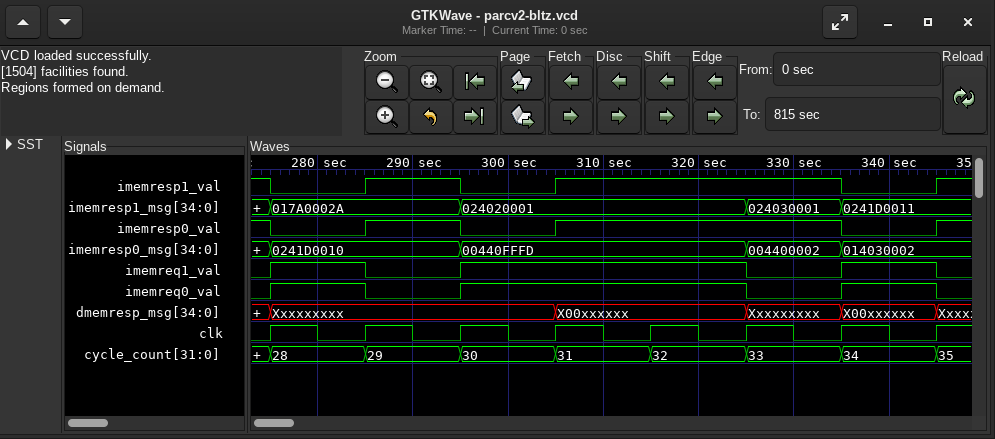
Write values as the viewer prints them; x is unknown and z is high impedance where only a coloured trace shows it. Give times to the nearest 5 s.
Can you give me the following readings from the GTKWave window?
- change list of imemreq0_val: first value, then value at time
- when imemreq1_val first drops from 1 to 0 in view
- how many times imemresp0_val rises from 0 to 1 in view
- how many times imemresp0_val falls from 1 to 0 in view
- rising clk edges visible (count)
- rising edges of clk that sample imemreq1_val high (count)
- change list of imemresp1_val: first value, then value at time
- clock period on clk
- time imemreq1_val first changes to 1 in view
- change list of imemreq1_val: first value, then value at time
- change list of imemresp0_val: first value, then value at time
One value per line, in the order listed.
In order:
0, 1 at 275 s, 0 at 285 s, 1 at 295 s, 0 at 325 s, 1 at 335 s, 0 at 345 s
285 s
3
3
8
5
1, 0 at 275 s, 1 at 285 s, 0 at 295 s, 1 at 305 s, 0 at 335 s, 1 at 345 s
10 s
275 s
0, 1 at 275 s, 0 at 285 s, 1 at 295 s, 0 at 325 s, 1 at 335 s, 0 at 345 s
1, 0 at 275 s, 1 at 285 s, 0 at 295 s, 1 at 305 s, 0 at 335 s, 1 at 345 s
